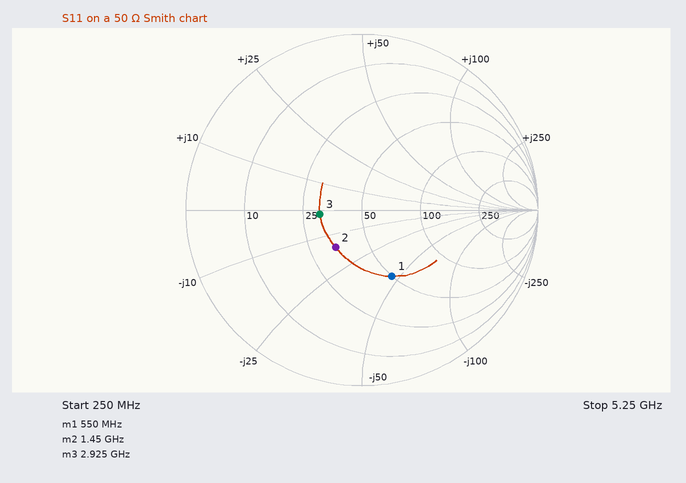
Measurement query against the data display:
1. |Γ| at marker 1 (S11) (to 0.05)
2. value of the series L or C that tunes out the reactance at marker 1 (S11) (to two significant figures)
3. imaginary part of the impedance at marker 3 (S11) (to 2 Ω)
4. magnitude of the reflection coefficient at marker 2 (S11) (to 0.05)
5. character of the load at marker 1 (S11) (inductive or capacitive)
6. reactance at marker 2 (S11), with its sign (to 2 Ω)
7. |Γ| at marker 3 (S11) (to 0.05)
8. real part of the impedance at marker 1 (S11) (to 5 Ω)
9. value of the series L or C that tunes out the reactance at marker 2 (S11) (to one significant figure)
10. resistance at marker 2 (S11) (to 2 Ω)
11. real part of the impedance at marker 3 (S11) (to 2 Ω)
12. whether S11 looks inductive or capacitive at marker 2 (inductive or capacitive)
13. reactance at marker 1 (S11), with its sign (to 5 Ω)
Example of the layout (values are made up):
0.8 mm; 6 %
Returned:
0.40; 13 nH; -2 Ω; 0.25; capacitive; -16 Ω; 0.25; 50 Ω; 2 nH; 34 Ω; 30 Ω; capacitive; -45 Ω
